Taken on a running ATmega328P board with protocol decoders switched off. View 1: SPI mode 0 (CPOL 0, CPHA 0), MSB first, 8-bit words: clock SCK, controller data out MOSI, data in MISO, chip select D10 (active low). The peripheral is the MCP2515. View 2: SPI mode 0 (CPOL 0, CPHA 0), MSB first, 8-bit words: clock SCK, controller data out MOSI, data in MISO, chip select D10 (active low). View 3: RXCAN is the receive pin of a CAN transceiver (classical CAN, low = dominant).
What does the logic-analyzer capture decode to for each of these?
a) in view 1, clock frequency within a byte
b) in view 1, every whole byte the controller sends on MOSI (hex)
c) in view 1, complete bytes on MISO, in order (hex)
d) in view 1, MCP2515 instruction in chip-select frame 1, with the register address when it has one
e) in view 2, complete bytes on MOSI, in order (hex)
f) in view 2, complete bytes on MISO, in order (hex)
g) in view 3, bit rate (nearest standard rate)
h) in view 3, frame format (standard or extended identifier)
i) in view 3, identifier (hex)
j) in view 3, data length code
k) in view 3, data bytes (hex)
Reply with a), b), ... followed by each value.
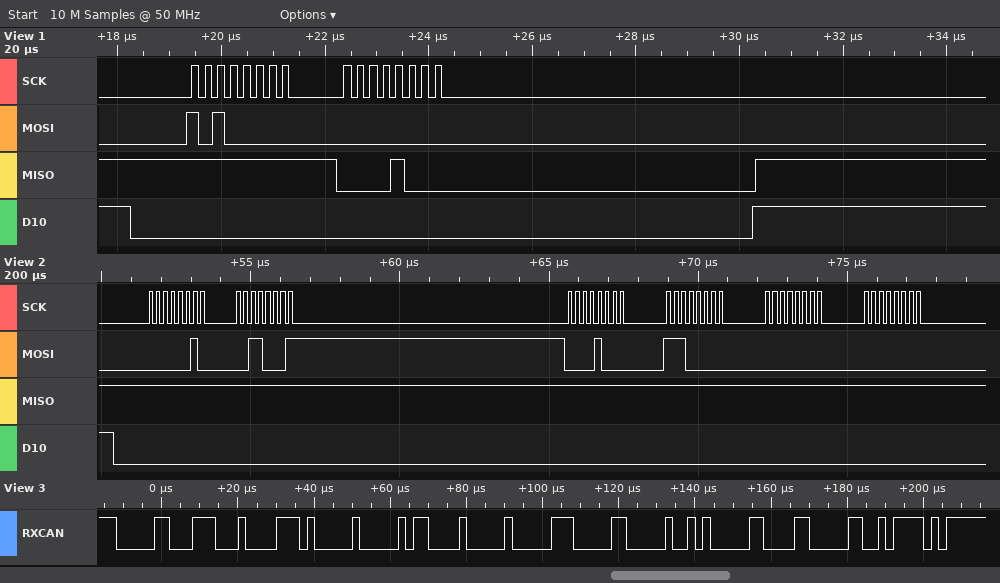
a) 4 MHz
b) A0 00
c) FF 08
d) READ STATUS
e) 0x02 0x31 0x08 0xE0 0x00 0x00
f) 0xFF 0xFF 0xFF 0xFF 0xFF 0xFF
g) 500 kbit/s
h) standard
i) 0x047
j) 8
k) 74 00 61 00 30 40 50 43
